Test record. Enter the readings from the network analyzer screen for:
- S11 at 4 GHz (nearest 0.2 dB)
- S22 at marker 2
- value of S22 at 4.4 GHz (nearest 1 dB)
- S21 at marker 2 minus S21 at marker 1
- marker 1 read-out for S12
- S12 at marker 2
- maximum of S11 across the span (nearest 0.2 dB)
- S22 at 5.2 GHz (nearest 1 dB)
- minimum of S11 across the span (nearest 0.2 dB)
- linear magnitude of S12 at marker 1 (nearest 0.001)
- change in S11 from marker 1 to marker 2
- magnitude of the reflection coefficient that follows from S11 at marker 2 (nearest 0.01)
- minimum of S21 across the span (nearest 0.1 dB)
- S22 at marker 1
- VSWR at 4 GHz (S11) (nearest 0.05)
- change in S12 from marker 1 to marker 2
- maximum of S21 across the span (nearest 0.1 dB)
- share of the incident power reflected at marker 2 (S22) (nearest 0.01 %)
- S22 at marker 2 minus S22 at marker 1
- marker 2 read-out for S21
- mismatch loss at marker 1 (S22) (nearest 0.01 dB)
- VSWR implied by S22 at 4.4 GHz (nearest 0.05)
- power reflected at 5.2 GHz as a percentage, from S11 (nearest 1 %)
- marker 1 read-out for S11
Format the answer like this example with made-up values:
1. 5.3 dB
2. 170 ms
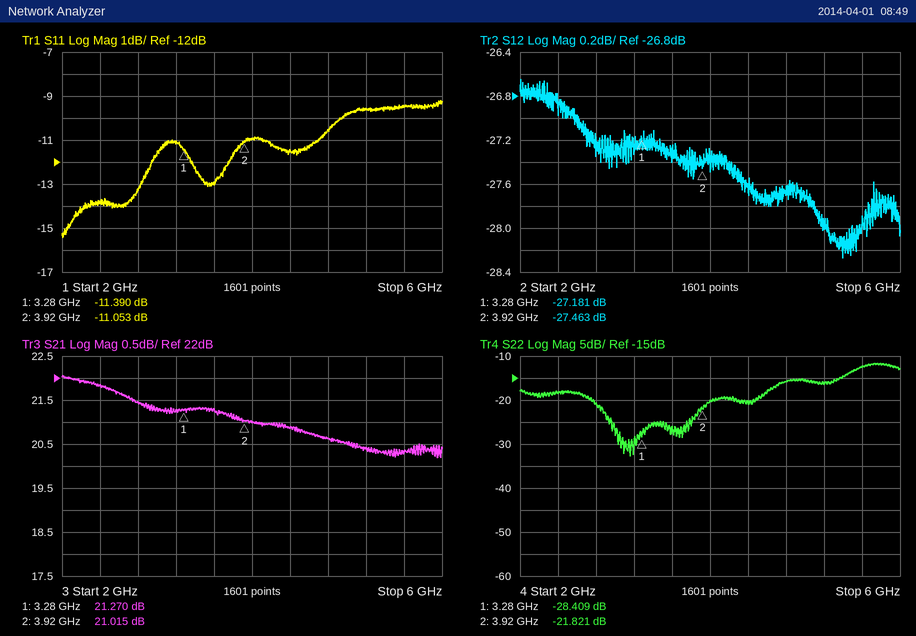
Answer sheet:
1. -11.0 dB
2. -21.821 dB
3. -20 dB
4. -0.255 dB
5. -27.181 dB
6. -27.463 dB
7. -9.2 dB
8. -16 dB
9. -15.4 dB
10. 0.044
11. 0.337 dB
12. 0.28
13. 20.2 dB
14. -28.409 dB
15. 1.80
16. -0.282 dB
17. 22.1 dB
18. 0.66 %
19. 6.588 dB
20. 21.015 dB
21. 0.01 dB
22. 1.20
23. 11 %
24. -11.390 dB
